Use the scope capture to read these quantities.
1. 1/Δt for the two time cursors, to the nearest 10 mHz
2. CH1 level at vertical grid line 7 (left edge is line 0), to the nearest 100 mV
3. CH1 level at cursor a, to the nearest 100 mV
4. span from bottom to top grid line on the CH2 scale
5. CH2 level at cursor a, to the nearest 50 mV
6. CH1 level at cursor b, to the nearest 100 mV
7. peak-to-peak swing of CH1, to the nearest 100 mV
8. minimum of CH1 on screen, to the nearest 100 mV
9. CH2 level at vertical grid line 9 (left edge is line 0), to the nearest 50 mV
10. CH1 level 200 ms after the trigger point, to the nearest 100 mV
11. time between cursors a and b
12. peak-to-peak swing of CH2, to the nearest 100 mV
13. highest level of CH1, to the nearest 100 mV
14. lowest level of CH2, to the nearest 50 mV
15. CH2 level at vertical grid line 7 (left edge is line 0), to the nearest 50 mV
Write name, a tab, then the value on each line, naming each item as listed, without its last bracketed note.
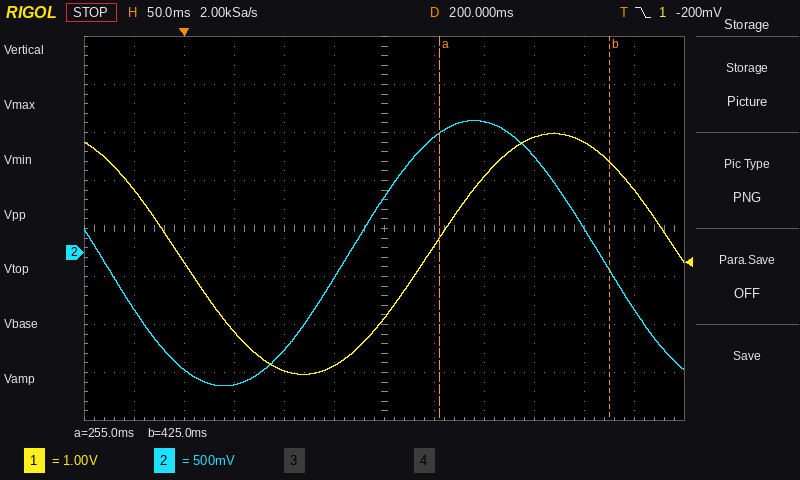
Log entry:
1/Δt for the two time cursors, to the nearest 10 mHz	5.88 Hz
CH1 level at vertical grid line 7 (left edge is line 0), to the nearest 100 mV	100 mV
CH1 level at cursor a, to the nearest 100 mV	300 mV
span from bottom to top grid line on the CH2 scale	4 V
CH2 level at cursor a, to the nearest 50 mV	1.25 V
CH1 level at cursor b, to the nearest 100 mV	1.9 V
peak-to-peak swing of CH1, to the nearest 100 mV	5.0 V
minimum of CH1 on screen, to the nearest 100 mV	-2.5 V
CH2 level at vertical grid line 9 (left edge is line 0), to the nearest 50 mV	1.00 V
CH1 level 200 ms after the trigger point, to the nearest 100 mV	-1.4 V
time between cursors a and b	170 ms
peak-to-peak swing of CH2, to the nearest 100 mV	2.80 V
highest level of CH1, to the nearest 100 mV	2.5 V
lowest level of CH2, to the nearest 50 mV	-1.40 V
CH2 level at vertical grid line 7 (left edge is line 0), to the nearest 50 mV	1.20 V
